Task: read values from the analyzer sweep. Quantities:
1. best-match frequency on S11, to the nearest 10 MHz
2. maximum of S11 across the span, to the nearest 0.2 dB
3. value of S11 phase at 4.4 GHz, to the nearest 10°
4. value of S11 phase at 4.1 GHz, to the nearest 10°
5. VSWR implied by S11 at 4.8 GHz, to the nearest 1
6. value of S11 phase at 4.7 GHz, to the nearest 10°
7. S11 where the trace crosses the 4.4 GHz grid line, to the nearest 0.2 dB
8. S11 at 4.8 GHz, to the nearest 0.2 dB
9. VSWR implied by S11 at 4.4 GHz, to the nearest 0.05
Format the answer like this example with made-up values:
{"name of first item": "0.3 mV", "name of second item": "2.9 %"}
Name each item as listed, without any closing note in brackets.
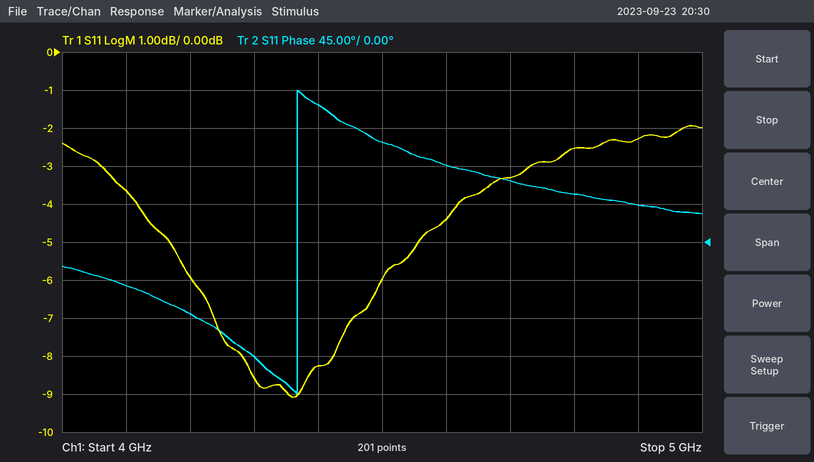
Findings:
{"best-match frequency on S11, to the nearest 10 MHz": "4.36 GHz", "maximum of S11 across the span, to the nearest 0.2 dB": "-2.0 dB", "value of S11 phase at 4.4 GHz, to the nearest 10°": "160°", "value of S11 phase at 4.1 GHz, to the nearest 10°": "-50°", "VSWR implied by S11 at 4.8 GHz, to the nearest 1": "7", "value of S11 phase at 4.7 GHz, to the nearest 10°": "70°", "S11 where the trace crosses the 4.4 GHz grid line, to the nearest 0.2 dB": "-8.2 dB", "S11 at 4.8 GHz, to the nearest 0.2 dB": "-2.6 dB", "VSWR implied by S11 at 4.4 GHz, to the nearest 0.05": "2.25"}
